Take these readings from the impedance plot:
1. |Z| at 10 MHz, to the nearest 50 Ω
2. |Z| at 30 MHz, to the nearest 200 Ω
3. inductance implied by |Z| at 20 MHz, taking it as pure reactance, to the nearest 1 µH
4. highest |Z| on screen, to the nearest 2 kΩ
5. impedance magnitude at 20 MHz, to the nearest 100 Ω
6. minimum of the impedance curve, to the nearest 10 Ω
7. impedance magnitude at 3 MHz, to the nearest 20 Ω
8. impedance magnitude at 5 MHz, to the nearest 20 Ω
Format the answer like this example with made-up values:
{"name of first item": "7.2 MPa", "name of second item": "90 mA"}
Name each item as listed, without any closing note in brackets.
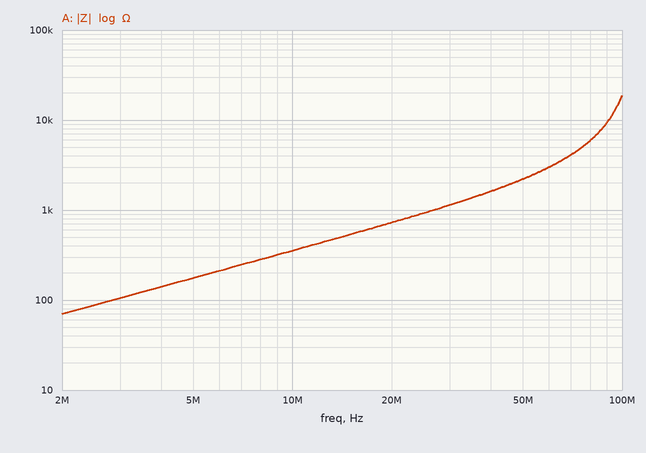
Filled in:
{"|Z| at 10 MHz, to the nearest 50 Ω": "350 Ω", "|Z| at 30 MHz, to the nearest 200 Ω": "1.2 kΩ", "inductance implied by |Z| at 20 MHz, taking it as pure reactance, to the nearest 1 µH": "6 µH", "highest |Z| on screen, to the nearest 2 kΩ": "18 kΩ", "impedance magnitude at 20 MHz, to the nearest 100 Ω": "700 Ω", "minimum of the impedance curve, to the nearest 10 Ω": "70 Ω", "impedance magnitude at 3 MHz, to the nearest 20 Ω": "100 Ω", "impedance magnitude at 5 MHz, to the nearest 20 Ω": "180 Ω"}
